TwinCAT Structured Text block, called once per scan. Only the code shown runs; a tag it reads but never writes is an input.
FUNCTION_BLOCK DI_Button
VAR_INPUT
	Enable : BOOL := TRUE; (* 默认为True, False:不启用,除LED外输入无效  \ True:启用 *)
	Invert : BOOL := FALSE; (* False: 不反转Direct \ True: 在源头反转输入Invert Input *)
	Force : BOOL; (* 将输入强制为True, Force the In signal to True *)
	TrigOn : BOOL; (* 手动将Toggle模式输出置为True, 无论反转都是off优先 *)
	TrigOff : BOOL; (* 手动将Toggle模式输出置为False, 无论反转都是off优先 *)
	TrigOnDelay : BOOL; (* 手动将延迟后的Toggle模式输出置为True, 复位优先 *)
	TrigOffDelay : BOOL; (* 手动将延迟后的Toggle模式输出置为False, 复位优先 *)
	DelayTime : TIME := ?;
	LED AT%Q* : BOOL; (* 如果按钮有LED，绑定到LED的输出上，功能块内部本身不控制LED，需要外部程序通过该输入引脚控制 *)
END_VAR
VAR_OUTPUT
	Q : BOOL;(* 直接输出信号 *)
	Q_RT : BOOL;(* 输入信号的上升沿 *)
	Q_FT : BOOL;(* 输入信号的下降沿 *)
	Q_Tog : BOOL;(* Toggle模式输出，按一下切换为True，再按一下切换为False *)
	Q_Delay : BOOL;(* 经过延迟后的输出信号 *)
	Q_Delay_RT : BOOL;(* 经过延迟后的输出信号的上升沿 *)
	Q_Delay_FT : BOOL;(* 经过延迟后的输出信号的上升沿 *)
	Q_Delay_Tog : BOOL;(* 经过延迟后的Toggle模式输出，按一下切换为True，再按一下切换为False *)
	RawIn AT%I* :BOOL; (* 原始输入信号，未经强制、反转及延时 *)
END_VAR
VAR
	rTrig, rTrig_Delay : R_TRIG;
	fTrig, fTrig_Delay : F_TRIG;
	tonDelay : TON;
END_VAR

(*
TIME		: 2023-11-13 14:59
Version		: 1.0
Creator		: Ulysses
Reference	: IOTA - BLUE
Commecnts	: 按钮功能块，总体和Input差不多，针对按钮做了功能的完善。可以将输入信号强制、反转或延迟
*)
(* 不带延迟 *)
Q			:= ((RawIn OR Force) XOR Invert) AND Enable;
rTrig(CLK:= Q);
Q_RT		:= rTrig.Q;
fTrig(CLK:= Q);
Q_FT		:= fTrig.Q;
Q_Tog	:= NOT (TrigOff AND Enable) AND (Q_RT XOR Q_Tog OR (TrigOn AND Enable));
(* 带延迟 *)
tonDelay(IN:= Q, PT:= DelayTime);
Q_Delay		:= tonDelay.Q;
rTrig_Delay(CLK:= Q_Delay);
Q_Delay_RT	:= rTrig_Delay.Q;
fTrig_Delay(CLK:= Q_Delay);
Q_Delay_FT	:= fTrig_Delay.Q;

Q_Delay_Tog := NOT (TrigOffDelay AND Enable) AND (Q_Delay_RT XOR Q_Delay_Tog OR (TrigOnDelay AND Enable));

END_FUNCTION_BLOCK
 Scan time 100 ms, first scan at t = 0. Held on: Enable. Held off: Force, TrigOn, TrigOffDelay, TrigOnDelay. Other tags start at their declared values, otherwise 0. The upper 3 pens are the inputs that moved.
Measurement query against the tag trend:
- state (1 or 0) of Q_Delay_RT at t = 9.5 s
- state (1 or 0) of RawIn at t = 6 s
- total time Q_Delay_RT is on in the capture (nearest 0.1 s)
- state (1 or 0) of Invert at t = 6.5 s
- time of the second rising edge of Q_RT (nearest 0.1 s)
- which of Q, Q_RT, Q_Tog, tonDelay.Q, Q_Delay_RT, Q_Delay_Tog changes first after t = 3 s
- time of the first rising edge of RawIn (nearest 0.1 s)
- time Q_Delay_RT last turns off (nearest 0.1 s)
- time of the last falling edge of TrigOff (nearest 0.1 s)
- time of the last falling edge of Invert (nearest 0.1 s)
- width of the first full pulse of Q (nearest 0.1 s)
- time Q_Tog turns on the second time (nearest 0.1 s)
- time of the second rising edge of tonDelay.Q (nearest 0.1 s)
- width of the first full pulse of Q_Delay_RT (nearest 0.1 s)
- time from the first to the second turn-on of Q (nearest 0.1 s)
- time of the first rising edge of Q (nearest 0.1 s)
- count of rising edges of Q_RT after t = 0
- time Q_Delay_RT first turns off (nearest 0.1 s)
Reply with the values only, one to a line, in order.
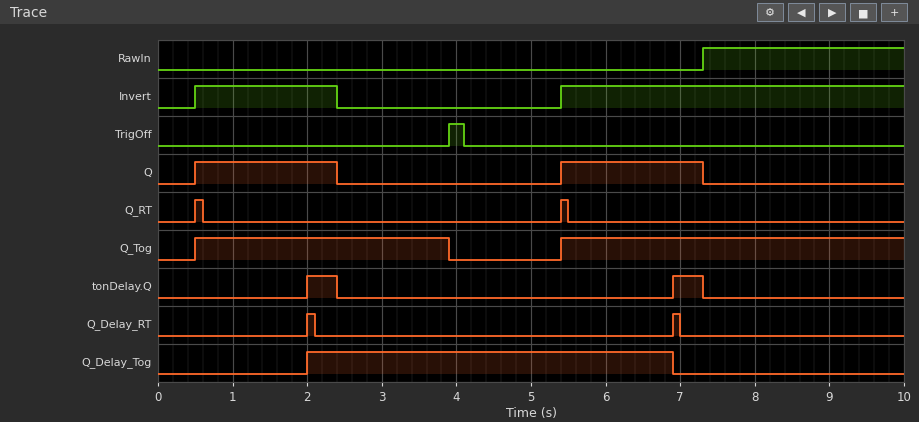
0
0
0.2 s
1
5.4 s
Q_Tog
7.3 s
7.0 s
4.1 s
2.4 s
1.9 s
5.4 s
6.9 s
0.1 s
4.9 s
0.5 s
2
2.1 s
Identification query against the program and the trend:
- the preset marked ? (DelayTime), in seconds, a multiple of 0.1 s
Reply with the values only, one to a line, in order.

1.5 s
